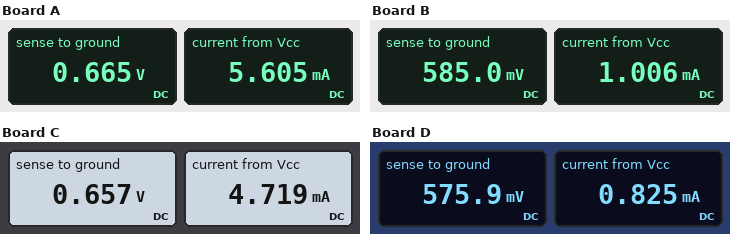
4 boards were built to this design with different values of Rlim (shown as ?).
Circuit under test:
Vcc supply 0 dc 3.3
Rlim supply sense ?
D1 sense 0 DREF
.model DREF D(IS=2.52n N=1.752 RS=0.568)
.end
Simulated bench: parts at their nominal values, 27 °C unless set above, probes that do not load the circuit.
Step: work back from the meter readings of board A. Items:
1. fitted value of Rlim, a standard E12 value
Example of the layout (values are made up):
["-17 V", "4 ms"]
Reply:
["470 Ω"]
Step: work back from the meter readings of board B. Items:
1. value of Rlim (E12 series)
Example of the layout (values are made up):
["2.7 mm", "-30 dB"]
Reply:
["2.7 kΩ"]
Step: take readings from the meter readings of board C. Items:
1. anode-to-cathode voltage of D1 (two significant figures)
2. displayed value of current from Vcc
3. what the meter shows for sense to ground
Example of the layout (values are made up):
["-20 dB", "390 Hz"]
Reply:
["660 mV", "4.719 mA", "0.657 V"]
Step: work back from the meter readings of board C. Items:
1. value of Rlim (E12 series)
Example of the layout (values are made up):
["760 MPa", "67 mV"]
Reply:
["560 Ω"]
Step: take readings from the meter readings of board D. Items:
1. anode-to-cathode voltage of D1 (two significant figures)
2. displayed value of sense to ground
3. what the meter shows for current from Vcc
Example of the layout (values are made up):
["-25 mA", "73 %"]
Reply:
["580 mV", "575.9 mV", "0.825 mA"]
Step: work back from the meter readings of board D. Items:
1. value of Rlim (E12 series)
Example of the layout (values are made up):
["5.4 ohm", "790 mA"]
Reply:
["3.3 kΩ"]
